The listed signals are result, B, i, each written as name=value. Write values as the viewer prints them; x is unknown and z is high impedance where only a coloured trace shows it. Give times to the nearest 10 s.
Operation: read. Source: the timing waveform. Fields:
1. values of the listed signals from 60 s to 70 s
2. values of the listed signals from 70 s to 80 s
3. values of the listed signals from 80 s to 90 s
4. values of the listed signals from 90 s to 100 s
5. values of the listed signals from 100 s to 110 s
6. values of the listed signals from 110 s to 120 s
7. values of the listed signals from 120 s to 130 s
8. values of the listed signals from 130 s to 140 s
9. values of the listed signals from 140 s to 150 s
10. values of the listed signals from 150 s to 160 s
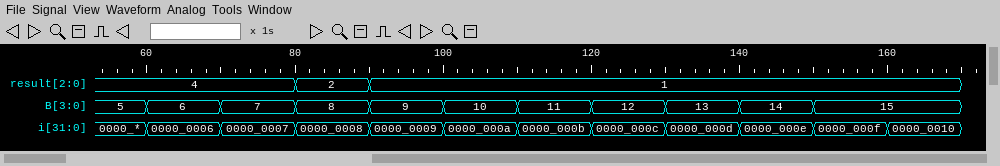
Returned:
result=4, B=6, i=0000_0006
result=4, B=7, i=0000_0007
result=2, B=8, i=0000_0008
result=1, B=9, i=0000_0009
result=1, B=10, i=0000_000a
result=1, B=11, i=0000_000b
result=1, B=12, i=0000_000c
result=1, B=13, i=0000_000d
result=1, B=14, i=0000_000e
result=1, B=15, i=0000_000f
